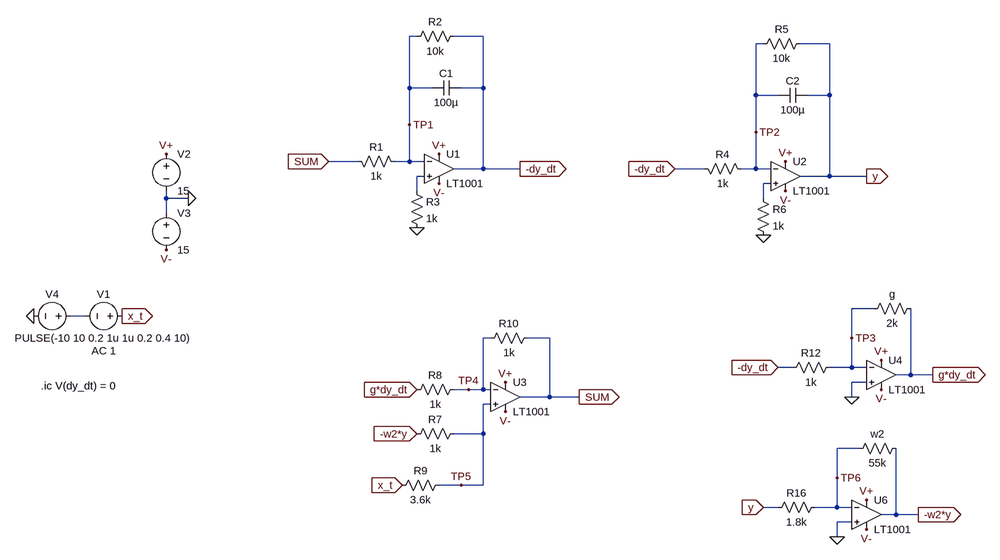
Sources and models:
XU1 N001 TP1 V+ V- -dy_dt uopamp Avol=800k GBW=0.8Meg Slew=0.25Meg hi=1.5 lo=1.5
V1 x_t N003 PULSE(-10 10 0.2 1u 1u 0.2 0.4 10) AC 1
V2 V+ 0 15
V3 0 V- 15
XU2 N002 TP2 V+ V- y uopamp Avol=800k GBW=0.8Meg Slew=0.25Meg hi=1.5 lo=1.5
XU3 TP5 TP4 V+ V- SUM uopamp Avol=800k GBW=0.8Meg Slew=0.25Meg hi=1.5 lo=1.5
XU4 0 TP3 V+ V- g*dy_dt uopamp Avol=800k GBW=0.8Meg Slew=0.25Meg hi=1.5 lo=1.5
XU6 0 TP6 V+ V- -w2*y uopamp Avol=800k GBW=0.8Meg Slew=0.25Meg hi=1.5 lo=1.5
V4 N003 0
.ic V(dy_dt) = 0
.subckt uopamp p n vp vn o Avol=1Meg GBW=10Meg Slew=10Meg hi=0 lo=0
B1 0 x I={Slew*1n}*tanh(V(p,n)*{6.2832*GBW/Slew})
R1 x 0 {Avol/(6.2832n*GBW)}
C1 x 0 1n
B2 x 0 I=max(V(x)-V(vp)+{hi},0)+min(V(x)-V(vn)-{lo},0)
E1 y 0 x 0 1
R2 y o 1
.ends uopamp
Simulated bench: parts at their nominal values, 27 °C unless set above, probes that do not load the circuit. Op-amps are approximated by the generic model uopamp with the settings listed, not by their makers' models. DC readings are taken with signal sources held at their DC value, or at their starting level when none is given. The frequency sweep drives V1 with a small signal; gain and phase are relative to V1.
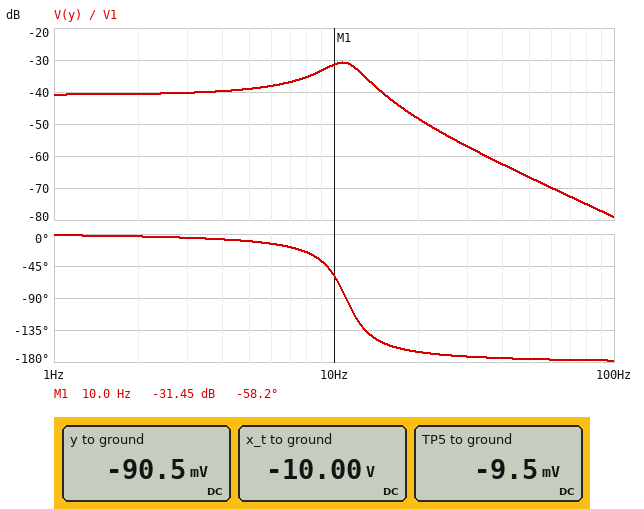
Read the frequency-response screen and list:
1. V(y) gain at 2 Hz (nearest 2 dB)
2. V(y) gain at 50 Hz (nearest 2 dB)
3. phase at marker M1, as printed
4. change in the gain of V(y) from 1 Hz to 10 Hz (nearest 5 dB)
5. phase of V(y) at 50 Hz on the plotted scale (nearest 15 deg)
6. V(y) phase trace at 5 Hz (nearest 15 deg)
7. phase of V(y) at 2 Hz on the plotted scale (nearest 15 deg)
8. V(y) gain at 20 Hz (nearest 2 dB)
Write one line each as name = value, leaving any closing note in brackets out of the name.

V(y) gain at 2 Hz = -40 dB
V(y) gain at 50 Hz = -66 dB
phase at marker M1, as printed = -58.2 deg
change in the gain of V(y) from 1 Hz to 10 Hz = 10 dB
phase of V(y) at 50 Hz on the plotted scale = -180 deg
V(y) phase trace at 5 Hz = -15 deg
phase of V(y) at 2 Hz on the plotted scale = 0 deg
V(y) gain at 20 Hz = -48 dB
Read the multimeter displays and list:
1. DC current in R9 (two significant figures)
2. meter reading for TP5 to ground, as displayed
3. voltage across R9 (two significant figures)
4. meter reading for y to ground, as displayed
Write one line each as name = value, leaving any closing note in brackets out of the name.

DC current in R9 = 2.8 mA
meter reading for TP5 to ground, as displayed = -9.5 mV
voltage across R9 = 10 V
meter reading for y to ground, as displayed = -90.5 mV
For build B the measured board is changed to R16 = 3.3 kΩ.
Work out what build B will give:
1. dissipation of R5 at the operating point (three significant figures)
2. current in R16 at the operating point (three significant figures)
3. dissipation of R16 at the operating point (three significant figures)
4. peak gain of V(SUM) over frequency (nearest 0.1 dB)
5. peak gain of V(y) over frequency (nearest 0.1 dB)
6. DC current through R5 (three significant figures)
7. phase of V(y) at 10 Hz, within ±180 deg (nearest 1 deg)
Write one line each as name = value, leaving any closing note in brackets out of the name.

dissipation of R5 at the operating point = 2.73 µW
current in R16 at the operating point = 50.1 µA
dissipation of R16 at the operating point = 8.28 µW
peak gain of V(SUM) over frequency = 0.3 dB
peak gain of V(y) over frequency = -28.1 dB
DC current through R5 = 16.5 µA
phase of V(y) at 10 Hz, within ±180 deg = -134 deg
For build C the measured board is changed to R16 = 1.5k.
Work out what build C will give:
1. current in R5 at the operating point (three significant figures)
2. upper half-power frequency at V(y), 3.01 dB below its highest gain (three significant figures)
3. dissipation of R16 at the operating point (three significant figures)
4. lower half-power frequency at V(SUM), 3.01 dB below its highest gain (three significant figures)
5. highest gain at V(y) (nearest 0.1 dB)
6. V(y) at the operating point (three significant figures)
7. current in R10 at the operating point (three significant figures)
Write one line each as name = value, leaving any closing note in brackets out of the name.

current in R5 at the operating point = 7.55 µA
upper half-power frequency at V(y), 3.01 dB below its highest gain = 13.5 Hz
dissipation of R16 at the operating point = 3.80 µW
lower half-power frequency at V(SUM), 3.01 dB below its highest gain = 10.8 Hz
highest gain at V(y) = -31.6 dB
V(y) at the operating point = -75.5 mV
current in R10 at the operating point = 7.17 µA
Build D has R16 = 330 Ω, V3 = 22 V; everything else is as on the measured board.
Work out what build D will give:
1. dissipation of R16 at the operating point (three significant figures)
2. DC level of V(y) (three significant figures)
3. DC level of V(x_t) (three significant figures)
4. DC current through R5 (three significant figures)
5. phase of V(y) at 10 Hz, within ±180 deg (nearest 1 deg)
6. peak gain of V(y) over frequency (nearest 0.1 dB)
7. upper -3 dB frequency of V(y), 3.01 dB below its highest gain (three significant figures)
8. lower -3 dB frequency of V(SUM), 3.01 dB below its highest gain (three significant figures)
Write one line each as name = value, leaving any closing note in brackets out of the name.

dissipation of R16 at the operating point = 840 nW
DC level of V(y) = -16.7 mV
DC level of V(x_t) = -10.0 V
DC current through R5 = 1.67 µA
phase of V(y) at 10 Hz, within ±180 deg = -3 deg
peak gain of V(y) over frequency = -37.9 dB
upper -3 dB frequency of V(y), 3.01 dB below its highest gain = 27.2 Hz
lower -3 dB frequency of V(SUM), 3.01 dB below its highest gain = 24.3 Hz
